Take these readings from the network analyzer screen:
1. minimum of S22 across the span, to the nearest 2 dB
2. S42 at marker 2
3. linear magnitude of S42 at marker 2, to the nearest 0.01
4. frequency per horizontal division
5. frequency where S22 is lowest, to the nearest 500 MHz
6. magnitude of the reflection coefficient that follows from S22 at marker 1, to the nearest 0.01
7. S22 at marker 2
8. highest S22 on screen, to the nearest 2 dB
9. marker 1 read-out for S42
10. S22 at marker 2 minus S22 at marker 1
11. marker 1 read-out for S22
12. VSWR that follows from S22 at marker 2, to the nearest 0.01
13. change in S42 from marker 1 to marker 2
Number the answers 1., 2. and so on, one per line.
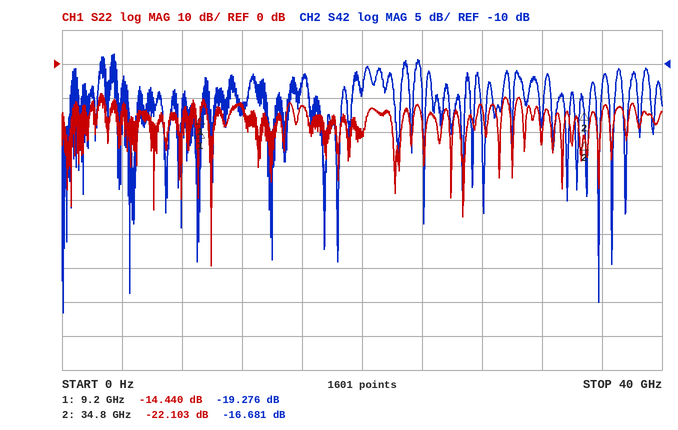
1. -60 dB
2. -16.681 dB
3. 0.15
4. 4 GHz
5. 10.0 GHz
6. 0.19
7. -22.103 dB
8. -8 dB
9. -19.276 dB
10. -7.663 dB
11. -14.440 dB
12. 1.17
13. 2.595 dB
